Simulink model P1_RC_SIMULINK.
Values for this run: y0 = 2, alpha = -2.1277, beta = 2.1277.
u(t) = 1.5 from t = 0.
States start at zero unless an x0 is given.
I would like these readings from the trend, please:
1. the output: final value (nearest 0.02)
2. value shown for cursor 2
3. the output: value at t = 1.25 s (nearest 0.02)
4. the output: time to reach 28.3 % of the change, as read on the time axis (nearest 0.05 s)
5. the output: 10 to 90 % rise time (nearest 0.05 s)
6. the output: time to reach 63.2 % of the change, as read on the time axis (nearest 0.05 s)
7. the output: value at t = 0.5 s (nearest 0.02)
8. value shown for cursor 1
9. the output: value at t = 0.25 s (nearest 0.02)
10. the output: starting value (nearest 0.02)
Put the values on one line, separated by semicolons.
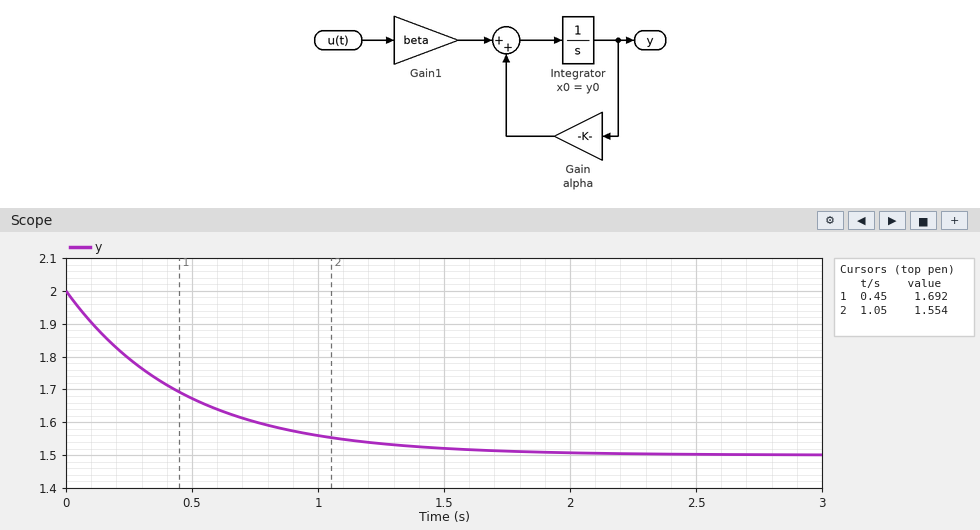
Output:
1.50; 1.554; 1.54; 0.15 s; 1.05 s; 0.45 s; 1.68; 1.692; 1.80; 2.00
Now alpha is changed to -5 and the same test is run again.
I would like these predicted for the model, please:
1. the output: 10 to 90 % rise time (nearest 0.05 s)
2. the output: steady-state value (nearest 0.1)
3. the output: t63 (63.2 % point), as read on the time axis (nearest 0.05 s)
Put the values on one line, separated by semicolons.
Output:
0.45 s; 0.6; 0.20 s
